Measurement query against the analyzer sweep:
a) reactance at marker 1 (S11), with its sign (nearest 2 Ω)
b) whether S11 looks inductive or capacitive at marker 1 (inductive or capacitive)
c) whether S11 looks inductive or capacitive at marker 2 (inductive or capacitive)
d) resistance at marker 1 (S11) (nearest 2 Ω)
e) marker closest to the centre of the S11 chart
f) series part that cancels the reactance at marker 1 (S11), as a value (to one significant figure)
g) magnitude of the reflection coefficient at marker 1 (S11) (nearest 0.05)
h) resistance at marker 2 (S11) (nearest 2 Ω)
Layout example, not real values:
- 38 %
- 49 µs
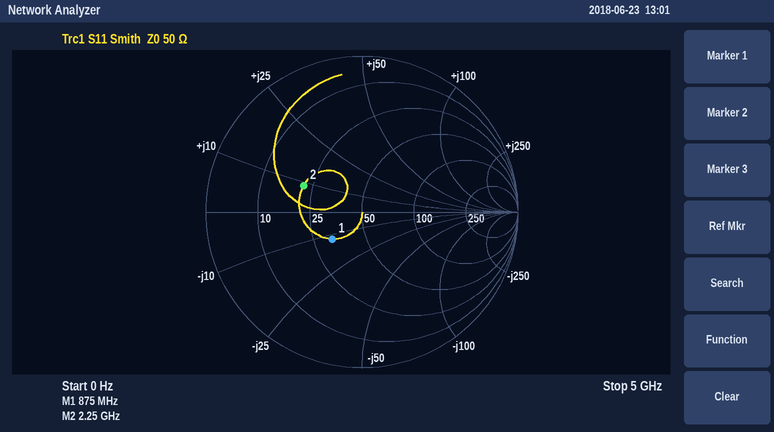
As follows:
- -12 Ω
- capacitive
- inductive
- 32 Ω
- marker 1
- 2 nH
- 0.25
- 22 Ω
